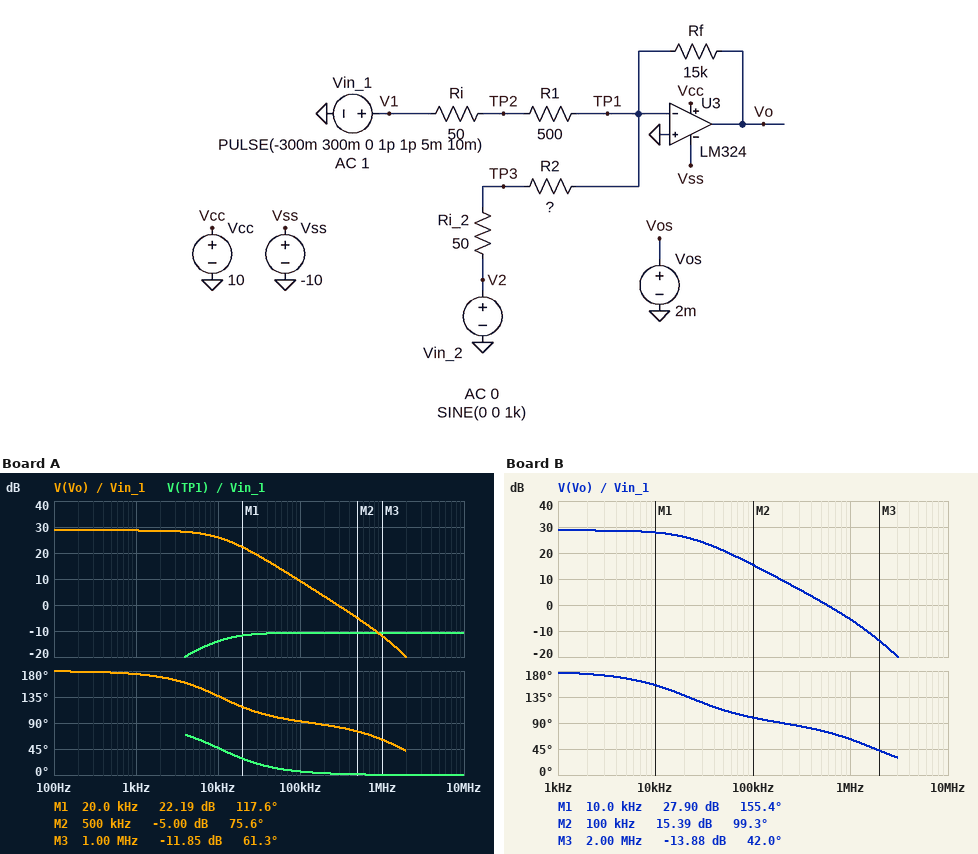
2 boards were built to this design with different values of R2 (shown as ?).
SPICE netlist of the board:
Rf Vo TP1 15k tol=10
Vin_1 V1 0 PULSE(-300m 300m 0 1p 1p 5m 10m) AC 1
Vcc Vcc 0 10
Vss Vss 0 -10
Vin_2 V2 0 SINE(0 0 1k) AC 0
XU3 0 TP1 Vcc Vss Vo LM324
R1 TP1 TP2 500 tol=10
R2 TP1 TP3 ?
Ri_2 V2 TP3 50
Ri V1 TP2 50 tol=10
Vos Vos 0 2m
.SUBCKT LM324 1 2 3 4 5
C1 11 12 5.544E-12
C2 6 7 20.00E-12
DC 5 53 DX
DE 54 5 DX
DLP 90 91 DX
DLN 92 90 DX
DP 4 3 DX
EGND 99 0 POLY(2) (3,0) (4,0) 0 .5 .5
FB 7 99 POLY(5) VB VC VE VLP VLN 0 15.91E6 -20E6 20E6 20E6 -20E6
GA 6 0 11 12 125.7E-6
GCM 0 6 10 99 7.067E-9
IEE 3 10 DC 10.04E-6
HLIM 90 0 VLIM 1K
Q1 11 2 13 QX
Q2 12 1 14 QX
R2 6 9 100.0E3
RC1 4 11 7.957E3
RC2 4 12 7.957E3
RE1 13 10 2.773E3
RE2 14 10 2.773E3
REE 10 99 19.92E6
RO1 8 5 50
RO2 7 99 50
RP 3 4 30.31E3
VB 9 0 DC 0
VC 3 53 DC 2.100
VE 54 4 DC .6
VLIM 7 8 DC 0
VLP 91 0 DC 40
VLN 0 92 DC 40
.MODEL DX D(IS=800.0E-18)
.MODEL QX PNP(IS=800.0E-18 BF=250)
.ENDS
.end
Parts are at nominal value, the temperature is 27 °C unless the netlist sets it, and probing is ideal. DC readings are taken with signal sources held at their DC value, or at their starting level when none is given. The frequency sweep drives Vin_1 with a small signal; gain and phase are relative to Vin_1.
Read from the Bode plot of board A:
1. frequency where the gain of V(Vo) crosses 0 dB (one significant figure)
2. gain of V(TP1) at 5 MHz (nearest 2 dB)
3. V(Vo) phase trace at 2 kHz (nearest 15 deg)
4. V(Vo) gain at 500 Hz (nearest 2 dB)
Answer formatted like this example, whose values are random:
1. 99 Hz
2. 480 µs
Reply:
1. 300 kHz
2. -10 dB
3. 165 deg
4. 28 dB
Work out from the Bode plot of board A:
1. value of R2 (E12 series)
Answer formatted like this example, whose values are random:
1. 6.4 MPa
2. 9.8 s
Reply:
1. 180 Ω
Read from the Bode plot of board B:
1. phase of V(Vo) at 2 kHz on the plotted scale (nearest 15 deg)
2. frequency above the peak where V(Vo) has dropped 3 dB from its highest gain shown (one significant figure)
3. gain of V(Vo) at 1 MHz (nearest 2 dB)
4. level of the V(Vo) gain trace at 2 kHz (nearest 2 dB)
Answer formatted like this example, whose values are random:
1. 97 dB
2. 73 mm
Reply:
1. 180 deg
2. 20 kHz
3. -6 dB
4. 28 dB
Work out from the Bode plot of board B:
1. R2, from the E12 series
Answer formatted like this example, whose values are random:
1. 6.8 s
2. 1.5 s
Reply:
1. 820 Ω
